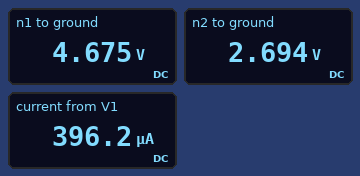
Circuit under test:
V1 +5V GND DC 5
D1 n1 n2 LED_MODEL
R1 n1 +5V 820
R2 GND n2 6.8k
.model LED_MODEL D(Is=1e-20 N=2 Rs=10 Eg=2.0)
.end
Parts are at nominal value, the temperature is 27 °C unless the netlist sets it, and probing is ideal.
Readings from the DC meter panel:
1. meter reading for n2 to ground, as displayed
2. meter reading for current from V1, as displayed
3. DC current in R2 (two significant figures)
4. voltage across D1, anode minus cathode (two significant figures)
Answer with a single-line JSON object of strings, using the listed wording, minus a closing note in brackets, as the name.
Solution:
{"meter reading for n2 to ground, as displayed": "2.694 V", "meter reading for current from V1, as displayed": "396.2 µA", "DC current in R2": "400 µA", "voltage across D1, anode minus cathode": "2.0 V"}
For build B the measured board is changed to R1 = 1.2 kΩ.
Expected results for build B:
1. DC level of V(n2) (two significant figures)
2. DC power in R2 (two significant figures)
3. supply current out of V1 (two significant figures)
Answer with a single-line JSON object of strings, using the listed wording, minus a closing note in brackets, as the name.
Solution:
{"DC level of V(n2)": "2.6 V", "DC power in R2": "970 µW", "supply current out of V1": "380 µA"}
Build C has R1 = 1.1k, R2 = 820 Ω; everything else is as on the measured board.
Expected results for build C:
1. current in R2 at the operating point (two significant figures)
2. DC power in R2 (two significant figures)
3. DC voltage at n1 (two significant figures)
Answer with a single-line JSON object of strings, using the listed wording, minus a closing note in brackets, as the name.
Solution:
{"current in R2 at the operating point": "1.5 mA", "DC power in R2": "1.9 mW", "DC voltage at n1": "3.3 V"}
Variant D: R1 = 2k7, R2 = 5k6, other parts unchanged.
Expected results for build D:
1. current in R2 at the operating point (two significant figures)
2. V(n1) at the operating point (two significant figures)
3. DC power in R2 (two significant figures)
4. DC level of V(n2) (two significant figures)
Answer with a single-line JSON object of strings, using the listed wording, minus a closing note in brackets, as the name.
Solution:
{"current in R2 at the operating point": "360 µA", "V(n1) at the operating point": "4.0 V", "DC power in R2": "740 µW", "DC level of V(n2)": "2.0 V"}
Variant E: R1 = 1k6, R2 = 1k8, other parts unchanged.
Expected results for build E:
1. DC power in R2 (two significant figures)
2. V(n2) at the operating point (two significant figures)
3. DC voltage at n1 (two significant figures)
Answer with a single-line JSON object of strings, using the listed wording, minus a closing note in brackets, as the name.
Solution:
{"DC power in R2": "1.4 mW", "V(n2) at the operating point": "1.6 V", "DC voltage at n1": "3.6 V"}
